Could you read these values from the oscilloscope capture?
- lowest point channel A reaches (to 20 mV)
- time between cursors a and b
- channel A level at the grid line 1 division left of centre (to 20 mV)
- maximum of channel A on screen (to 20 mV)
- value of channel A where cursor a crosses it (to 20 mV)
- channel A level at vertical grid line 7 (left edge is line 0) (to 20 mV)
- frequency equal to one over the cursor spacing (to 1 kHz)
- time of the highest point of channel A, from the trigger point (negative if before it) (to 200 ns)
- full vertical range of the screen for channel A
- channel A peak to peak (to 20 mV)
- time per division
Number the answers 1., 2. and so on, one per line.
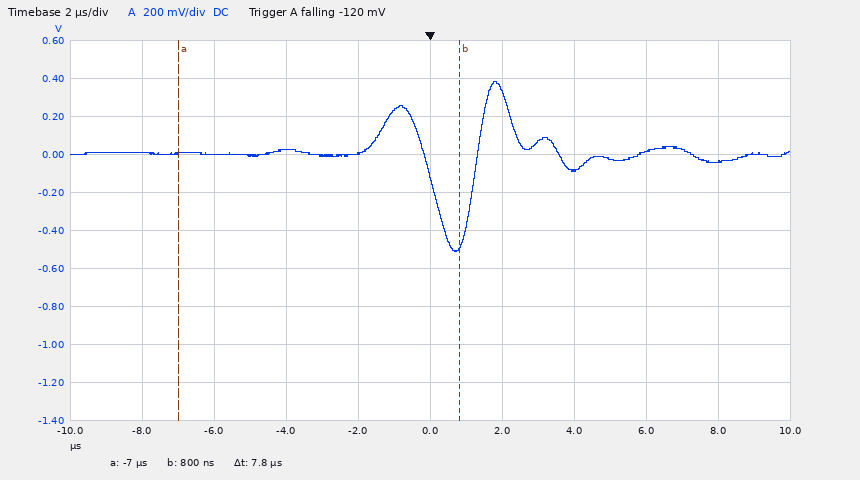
1. -520 mV
2. 7.8 µs
3. 0 mV
4. 380 mV
5. 0 mV
6. -80 mV
7. 128 kHz
8. +1.8 µs
9. 2 V
10. 900 mV
11. 2 µs
